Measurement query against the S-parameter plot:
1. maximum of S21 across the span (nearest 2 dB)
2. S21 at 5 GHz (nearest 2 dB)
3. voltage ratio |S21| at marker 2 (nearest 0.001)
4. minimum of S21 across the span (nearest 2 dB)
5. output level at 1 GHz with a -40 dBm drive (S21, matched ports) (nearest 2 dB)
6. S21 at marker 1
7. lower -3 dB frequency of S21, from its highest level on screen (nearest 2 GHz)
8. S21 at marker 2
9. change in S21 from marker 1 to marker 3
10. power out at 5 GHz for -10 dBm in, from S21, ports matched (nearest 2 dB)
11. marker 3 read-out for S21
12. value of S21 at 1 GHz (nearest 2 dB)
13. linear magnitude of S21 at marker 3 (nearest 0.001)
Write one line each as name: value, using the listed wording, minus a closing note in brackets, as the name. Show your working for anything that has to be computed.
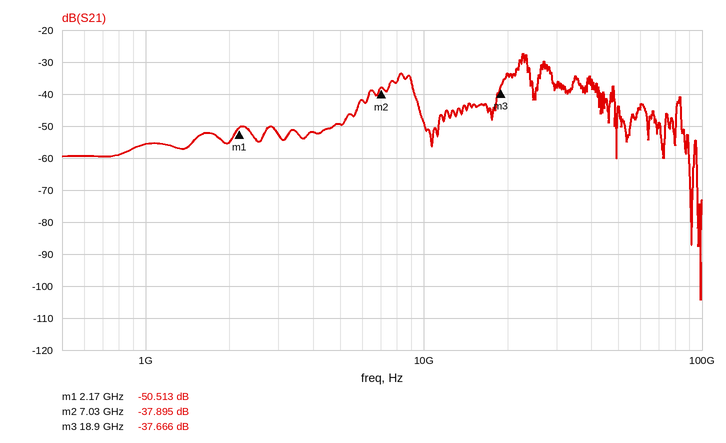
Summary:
maximum of S21 across the span: -28 dB
S21 at 5 GHz: -50 dB
voltage ratio |S21| at marker 2: 10^(-37.895/20) ≈ 0.013
minimum of S21 across the span: -104 dB
output level at 1 GHz with a -40 dBm drive (S21, matched ports): -40 dBm + (-56 dB) = -96 dBm
S21 at marker 1: -50.513 dB
lower -3 dB frequency of S21, from its highest level on screen: 22 GHz
S21 at marker 2: -37.895 dB
change in S21 from marker 1 to marker 3: -37.666 − (-50.513) = 12.847 dB
power out at 5 GHz for -10 dBm in, from S21, ports matched: -10 dBm + (-50 dB) = -60 dBm
marker 3 read-out for S21: -37.666 dB
value of S21 at 1 GHz: -56 dB
linear magnitude of S21 at marker 3: 10^(-37.666/20) ≈ 0.013
